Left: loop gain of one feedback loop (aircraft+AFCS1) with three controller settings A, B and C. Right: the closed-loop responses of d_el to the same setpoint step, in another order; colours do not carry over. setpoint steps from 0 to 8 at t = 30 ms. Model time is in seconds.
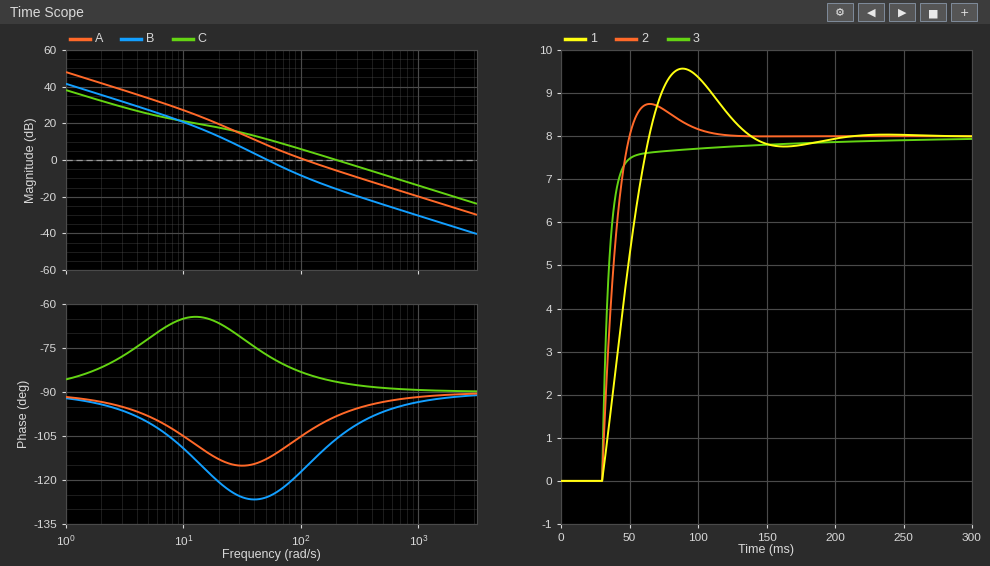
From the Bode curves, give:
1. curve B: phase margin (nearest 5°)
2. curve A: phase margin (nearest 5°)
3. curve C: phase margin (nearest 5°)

55°
75°
95°
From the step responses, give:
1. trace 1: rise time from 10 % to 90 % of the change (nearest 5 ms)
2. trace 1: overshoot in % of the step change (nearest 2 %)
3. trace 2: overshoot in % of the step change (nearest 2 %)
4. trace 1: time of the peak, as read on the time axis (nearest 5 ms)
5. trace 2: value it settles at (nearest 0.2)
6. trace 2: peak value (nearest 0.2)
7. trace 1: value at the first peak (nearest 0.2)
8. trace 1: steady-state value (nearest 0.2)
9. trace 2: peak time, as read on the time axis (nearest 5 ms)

25 ms
20 %
10 %
90 ms
8.0
8.8
9.6
8.0
65 ms
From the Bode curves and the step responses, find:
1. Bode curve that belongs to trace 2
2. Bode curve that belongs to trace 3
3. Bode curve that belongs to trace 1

A
C
B
